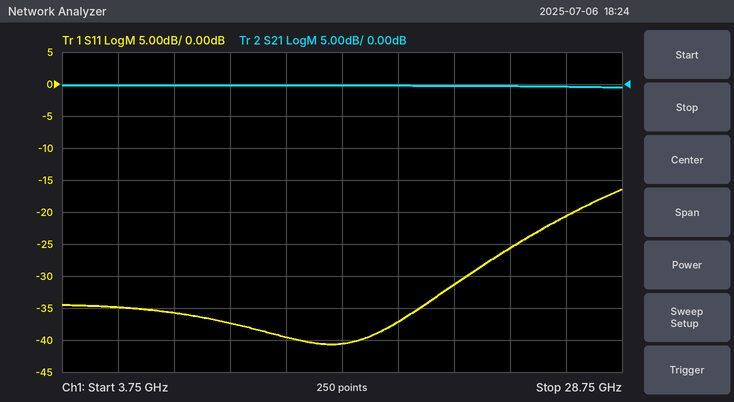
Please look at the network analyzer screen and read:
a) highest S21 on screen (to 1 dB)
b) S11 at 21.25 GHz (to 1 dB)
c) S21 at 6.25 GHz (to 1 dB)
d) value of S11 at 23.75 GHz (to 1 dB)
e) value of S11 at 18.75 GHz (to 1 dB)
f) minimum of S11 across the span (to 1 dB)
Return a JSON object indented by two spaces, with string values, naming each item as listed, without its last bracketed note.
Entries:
{
  "highest S21 on screen": "0 dB",
  "S11 at 21.25 GHz": "-31 dB",
  "S21 at 6.25 GHz": "0 dB",
  "value of S11 at 23.75 GHz": "-26 dB",
  "value of S11 at 18.75 GHz": "-37 dB",
  "minimum of S11 across the span": "-41 dB"
}
